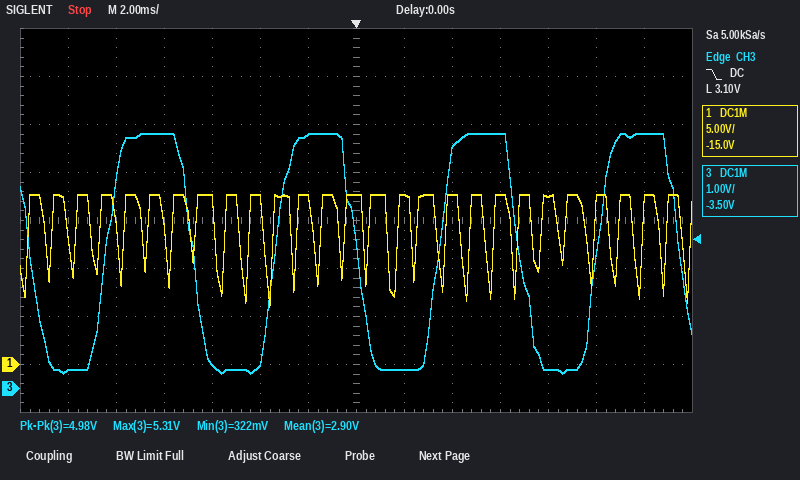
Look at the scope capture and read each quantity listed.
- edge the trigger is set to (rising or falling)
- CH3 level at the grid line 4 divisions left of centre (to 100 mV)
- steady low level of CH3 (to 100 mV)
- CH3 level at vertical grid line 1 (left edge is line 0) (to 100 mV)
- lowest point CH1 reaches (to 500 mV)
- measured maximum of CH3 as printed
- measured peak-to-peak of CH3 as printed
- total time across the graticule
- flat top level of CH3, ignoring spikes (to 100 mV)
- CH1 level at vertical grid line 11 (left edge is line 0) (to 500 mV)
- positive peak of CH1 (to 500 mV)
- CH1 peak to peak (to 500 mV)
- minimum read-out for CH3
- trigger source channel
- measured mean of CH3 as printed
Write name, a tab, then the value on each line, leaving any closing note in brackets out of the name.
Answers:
edge the trigger is set to	falling
CH3 level at the grid line 4 divisions left of centre	5.3 V
steady low level of CH3	400 mV
CH3 level at vertical grid line 1 (left edge is line 0)	400 mV
lowest point CH1 reaches	6.0 V
measured maximum of CH3 as printed	5.31 V
measured peak-to-peak of CH3 as printed	4.98 V
total time across the graticule	28 ms
flat top level of CH3, ignoring spikes	5.3 V
CH1 level at vertical grid line 11 (left edge is line 0)	17.5 V
positive peak of CH1	17.5 V
CH1 peak to peak	11.5 V
minimum read-out for CH3	322 mV
trigger source channel	CH3
measured mean of CH3 as printed	2.90 V
